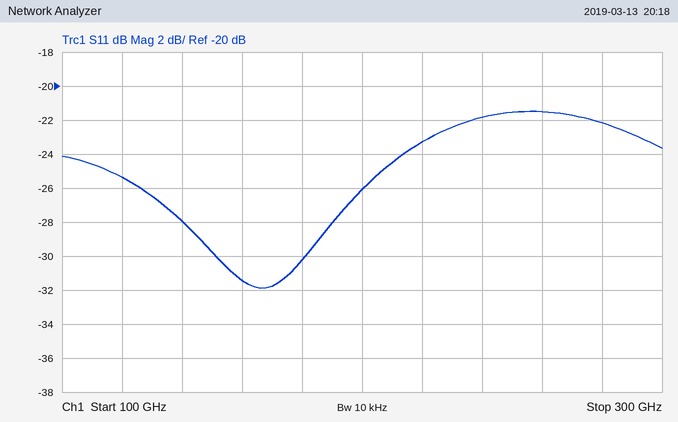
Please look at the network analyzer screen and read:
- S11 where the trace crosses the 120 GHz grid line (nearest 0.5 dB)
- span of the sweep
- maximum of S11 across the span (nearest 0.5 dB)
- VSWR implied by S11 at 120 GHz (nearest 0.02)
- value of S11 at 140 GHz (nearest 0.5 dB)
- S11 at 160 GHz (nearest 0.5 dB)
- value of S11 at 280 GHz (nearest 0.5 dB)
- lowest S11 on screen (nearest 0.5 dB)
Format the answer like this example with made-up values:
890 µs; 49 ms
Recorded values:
-25.5 dB; 200 GHz; -21.5 dB; 1.12; -28.0 dB; -31.5 dB; -22.0 dB; -32.0 dB
